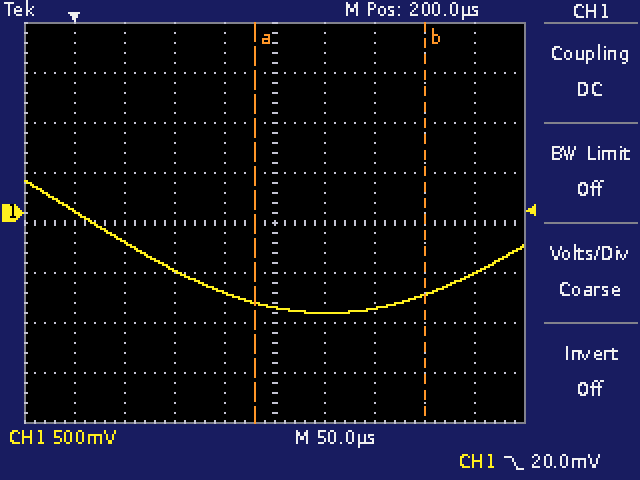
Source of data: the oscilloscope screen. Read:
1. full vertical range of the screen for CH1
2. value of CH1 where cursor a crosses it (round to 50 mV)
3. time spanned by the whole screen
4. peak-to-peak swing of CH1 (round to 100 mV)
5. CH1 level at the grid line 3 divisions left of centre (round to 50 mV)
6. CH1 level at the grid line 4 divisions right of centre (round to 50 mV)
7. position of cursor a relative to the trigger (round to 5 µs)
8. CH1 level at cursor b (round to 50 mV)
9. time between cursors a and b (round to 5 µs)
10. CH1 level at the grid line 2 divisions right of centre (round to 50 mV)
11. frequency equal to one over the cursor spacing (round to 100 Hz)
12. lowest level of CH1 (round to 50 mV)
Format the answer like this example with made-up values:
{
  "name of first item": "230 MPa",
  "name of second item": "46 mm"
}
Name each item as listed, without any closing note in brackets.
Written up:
{
  "full vertical range of the screen for CH1": "4 V",
  "value of CH1 where cursor a crosses it": "-900 mV",
  "time spanned by the whole screen": "500 µs",
  "peak-to-peak swing of CH1": "1.30 V",
  "CH1 level at the grid line 3 divisions left of centre": "-300 mV",
  "CH1 level at the grid line 4 divisions right of centre": "-600 mV",
  "position of cursor a relative to the trigger": "+180 µs",
  "CH1 level at cursor b": "-800 mV",
  "time between cursors a and b": "170 µs",
  "CH1 level at the grid line 2 divisions right of centre": "-950 mV",
  "frequency equal to one over the cursor spacing": "5.9 kHz",
  "lowest level of CH1": "-1.00 V"
}
